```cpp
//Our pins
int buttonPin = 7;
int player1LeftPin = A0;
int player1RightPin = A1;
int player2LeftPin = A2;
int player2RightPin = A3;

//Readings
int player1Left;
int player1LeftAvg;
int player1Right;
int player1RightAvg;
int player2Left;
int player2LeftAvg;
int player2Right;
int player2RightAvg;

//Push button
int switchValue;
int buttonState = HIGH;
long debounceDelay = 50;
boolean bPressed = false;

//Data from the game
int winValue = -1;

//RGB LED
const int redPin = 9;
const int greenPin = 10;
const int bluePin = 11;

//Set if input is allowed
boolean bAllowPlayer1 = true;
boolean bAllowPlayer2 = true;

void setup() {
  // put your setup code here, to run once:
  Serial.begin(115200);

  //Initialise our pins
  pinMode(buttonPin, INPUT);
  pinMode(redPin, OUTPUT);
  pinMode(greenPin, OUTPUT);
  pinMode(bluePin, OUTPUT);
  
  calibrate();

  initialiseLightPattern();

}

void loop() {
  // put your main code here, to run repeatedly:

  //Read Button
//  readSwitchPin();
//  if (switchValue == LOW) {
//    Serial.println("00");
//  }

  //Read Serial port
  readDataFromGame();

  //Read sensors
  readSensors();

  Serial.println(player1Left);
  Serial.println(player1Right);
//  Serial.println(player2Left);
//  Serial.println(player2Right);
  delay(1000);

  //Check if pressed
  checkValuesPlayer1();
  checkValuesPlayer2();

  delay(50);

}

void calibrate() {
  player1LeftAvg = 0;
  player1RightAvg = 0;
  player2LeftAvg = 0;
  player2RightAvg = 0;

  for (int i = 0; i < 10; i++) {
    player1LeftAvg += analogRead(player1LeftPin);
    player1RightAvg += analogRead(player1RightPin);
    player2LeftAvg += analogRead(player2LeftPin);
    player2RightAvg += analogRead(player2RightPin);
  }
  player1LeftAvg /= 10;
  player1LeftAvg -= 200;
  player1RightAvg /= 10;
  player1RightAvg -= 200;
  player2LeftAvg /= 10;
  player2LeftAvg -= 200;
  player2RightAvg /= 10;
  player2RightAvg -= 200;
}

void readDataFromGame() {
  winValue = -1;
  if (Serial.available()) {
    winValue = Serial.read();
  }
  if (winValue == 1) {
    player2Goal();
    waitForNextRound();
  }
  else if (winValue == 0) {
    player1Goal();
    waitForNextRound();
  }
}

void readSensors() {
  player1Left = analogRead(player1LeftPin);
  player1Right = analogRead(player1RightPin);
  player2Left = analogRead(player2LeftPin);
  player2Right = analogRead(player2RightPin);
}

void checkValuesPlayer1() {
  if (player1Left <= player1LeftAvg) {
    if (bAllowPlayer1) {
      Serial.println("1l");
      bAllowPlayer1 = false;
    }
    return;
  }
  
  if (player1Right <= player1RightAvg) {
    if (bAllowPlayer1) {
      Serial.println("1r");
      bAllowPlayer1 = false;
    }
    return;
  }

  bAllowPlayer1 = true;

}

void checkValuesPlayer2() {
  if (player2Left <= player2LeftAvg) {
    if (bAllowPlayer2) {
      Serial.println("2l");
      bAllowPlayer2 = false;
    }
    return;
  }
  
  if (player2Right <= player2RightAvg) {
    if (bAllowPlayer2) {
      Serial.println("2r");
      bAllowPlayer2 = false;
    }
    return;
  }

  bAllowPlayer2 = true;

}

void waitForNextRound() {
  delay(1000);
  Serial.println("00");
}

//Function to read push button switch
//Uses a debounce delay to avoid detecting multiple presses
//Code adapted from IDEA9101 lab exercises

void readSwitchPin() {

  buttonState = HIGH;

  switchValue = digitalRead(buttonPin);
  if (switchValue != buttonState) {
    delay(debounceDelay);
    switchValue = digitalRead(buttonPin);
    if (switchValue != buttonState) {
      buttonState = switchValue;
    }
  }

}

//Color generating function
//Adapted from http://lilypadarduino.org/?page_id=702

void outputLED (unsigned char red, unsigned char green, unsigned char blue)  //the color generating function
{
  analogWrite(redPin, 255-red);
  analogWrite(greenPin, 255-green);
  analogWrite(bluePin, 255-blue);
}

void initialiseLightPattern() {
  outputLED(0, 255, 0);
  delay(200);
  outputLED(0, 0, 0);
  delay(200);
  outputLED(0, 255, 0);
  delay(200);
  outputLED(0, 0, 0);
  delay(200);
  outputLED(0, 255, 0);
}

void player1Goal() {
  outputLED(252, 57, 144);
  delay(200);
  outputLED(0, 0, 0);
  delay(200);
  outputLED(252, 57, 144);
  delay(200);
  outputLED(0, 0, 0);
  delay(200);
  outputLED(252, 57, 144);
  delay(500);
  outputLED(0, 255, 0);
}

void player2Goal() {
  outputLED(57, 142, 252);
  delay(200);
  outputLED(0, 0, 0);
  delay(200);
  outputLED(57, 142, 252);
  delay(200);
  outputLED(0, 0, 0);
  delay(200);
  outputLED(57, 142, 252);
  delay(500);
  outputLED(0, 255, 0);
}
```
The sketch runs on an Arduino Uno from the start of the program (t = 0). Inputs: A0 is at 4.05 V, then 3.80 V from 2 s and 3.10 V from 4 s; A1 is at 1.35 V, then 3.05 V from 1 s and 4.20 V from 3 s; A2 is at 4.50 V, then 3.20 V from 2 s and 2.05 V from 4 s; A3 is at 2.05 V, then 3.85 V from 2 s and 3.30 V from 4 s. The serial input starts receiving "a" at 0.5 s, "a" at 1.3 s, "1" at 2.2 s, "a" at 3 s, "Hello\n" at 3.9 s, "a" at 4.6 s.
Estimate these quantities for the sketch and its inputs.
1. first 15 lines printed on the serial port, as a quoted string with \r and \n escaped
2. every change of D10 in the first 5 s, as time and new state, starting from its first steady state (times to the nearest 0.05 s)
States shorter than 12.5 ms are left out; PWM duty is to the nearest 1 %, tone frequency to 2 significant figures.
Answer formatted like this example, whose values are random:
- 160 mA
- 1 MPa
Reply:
- "829\r\n276\r\n829\r\n624\r\n778\r\n624\r\n2l\r\n778\r\n860\r\n634\r\n860\r\n634\r\n860\r\n634\r\n860\r\n"
- 0 s low; 0.2 s high; 0.4 s low; 0.6 s high; 0.8 s low
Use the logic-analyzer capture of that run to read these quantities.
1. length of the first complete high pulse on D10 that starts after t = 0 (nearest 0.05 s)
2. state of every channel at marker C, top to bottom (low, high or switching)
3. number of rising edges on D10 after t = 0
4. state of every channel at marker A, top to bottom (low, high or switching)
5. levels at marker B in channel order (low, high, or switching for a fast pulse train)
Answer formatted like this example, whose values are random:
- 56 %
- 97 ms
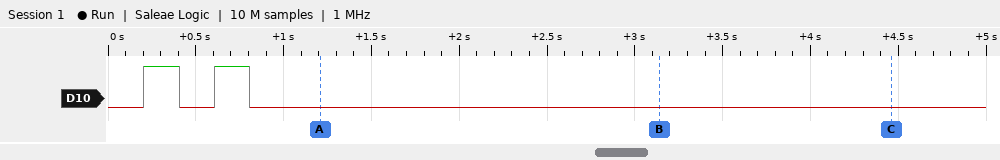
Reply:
- 0.20 s
- D10 low
- 2
- D10 low
- D10 low
